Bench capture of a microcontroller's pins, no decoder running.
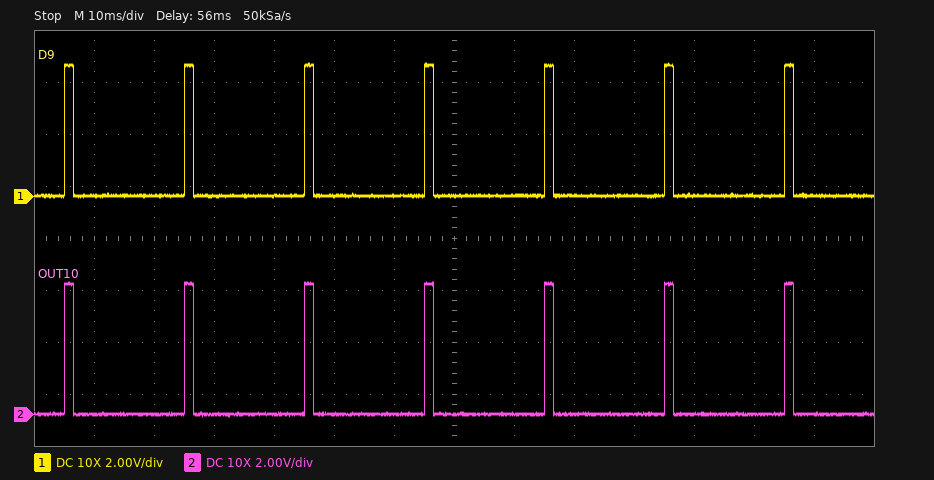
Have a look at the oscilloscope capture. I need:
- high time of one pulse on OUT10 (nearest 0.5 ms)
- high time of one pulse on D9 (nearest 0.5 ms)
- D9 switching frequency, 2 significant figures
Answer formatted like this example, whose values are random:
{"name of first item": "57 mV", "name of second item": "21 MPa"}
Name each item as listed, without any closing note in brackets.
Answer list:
{"high time of one pulse on OUT10": "1.5 ms", "high time of one pulse on D9": "1.5 ms", "D9 switching frequency, 2 significant figures": "50 Hz"}
